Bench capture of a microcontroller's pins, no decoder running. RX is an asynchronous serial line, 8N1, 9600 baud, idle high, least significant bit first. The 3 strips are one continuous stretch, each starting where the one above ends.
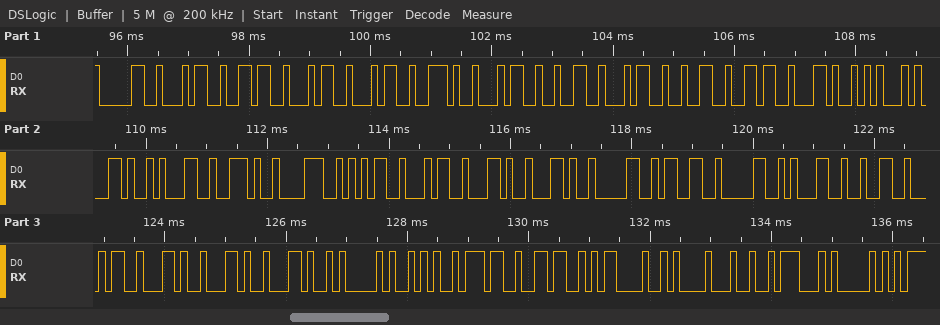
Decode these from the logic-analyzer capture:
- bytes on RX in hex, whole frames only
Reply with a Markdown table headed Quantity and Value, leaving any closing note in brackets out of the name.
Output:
| Quantity | Value |
|---|---|
| bytes on RX in hex, whole frames only | 30 34 36 34 34 2E 34 32 34 32 36 2C 45 2C 31 2E 38 35 34 2C 2C 30 33 30 31 32 34 2C 2C 2C 41 2A 37 36 0D 0A 24 47 50 |
